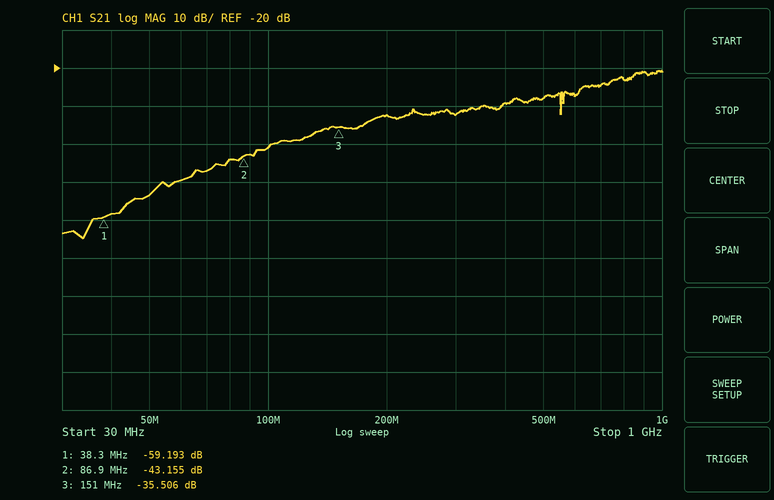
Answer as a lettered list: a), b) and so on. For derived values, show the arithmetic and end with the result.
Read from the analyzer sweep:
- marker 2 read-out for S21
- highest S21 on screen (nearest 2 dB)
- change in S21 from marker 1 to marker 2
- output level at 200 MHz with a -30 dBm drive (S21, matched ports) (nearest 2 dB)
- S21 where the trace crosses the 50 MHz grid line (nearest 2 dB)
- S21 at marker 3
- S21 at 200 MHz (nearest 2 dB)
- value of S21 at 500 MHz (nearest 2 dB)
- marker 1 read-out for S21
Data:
a) -43.155 dB
b) -20 dB
c) -43.155 − (-59.193) = 16.038 dB
d) -30 dBm + (-32 dB) = -62 dBm
e) -54 dB
f) -35.506 dB
g) -32 dB
h) -28 dB
i) -59.193 dB
